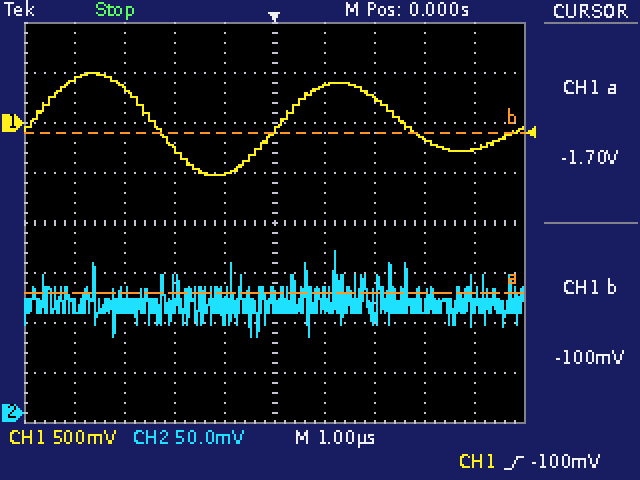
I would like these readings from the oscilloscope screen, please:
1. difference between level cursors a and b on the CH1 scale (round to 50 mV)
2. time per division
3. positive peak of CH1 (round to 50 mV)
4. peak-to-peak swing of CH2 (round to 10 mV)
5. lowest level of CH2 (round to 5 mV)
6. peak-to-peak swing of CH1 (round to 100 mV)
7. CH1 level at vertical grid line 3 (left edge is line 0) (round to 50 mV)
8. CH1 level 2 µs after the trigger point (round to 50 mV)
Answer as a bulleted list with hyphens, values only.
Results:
- 1.60 V
- 1 µs
- 500 mV
- 90 mV
- 75 mV
- 1.00 V
- -250 mV
- 250 mV
